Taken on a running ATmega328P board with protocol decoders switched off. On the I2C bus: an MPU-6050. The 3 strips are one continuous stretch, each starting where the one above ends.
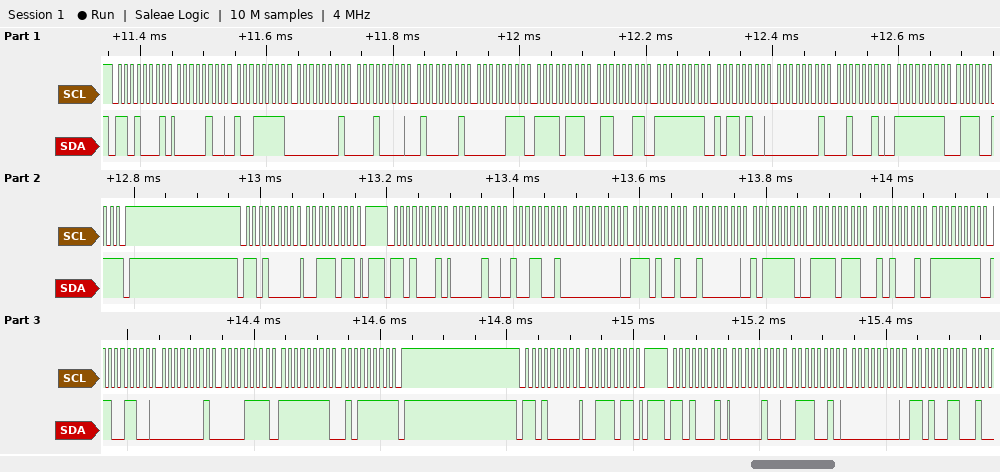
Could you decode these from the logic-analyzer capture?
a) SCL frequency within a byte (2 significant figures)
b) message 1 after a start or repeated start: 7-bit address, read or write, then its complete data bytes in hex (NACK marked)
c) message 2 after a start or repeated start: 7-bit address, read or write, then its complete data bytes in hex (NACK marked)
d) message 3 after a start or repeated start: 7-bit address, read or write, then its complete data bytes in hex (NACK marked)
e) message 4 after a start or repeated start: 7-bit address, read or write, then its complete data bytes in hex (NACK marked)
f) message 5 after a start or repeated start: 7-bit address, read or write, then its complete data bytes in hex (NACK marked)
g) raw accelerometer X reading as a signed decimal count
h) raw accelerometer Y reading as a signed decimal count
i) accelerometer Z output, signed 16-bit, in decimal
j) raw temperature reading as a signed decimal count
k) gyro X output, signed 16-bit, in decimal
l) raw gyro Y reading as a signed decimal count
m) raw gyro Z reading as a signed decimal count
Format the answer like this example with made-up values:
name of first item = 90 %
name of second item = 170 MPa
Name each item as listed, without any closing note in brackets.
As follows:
SCL frequency within a byte = 100 kHz
message 1 after a start or repeated start: 7-bit address, read or write, then its complete data bytes in hex = 0x68 read: 04 9F 01 10 41 07 F7 63 FF B4 01 22 FF 73 NACK
message 2 after a start or repeated start: 7-bit address, read or write, then its complete data bytes in hex = 0x68 write: 3B
message 3 after a start or repeated start: 7-bit address, read or write, then its complete data bytes in hex = 0x68 read: 04 99 00 E9 40 BE F7 51 FF CC 01 0F FF 5F NACK
message 4 after a start or repeated start: 7-bit address, read or write, then its complete data bytes in hex = 0x68 write: 3B
message 5 after a start or repeated start: 7-bit address, read or write, then its complete data bytes in hex = 0x68 read: 04 72 00 D3
raw accelerometer X reading as a signed decimal count = 1177
raw accelerometer Y reading as a signed decimal count = 233
accelerometer Z output, signed 16-bit, in decimal = 16574
raw temperature reading as a signed decimal count = -2223
gyro X output, signed 16-bit, in decimal = -52
raw gyro Y reading as a signed decimal count = 271
raw gyro Z reading as a signed decimal count = -161
